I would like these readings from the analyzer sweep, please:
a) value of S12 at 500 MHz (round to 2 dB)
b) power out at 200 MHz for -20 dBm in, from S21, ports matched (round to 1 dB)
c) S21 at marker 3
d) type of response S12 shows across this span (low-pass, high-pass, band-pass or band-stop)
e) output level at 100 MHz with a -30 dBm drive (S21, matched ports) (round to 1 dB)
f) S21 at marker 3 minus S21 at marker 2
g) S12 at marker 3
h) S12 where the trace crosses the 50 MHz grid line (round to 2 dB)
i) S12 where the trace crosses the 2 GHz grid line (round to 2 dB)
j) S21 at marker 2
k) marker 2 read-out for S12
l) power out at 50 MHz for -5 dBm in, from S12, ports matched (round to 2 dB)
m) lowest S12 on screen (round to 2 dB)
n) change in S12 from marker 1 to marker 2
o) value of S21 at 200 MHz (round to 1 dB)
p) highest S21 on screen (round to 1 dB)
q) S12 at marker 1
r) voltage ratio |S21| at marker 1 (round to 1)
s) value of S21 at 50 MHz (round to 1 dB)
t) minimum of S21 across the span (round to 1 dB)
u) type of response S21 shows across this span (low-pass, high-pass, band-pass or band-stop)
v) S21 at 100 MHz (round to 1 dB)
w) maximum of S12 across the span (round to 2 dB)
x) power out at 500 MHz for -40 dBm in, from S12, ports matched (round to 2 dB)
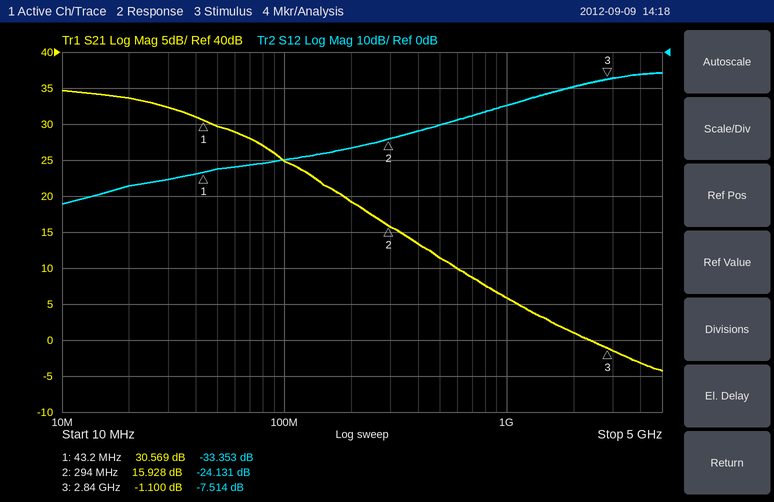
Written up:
-20 dB
-1 dBm
-1.100 dB
high-pass
-5 dBm
-17.028 dB
-7.514 dB
-32 dB
-10 dB
15.928 dB
-24.131 dB
-38 dBm
-42 dB
9.222 dB
19 dB
35 dB
-33.353 dB
34
30 dB
-4 dB
low-pass
25 dB
-6 dB
-60 dBm
